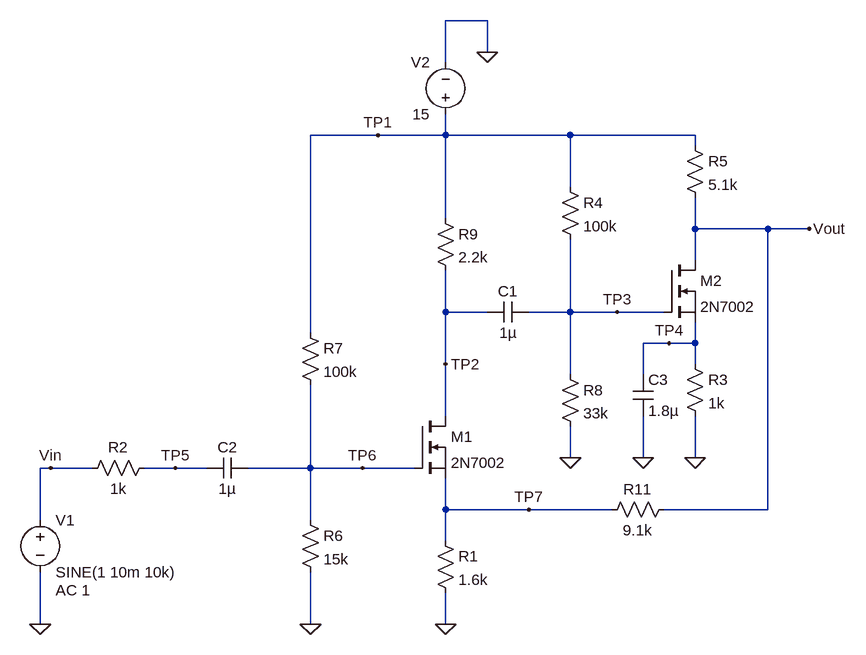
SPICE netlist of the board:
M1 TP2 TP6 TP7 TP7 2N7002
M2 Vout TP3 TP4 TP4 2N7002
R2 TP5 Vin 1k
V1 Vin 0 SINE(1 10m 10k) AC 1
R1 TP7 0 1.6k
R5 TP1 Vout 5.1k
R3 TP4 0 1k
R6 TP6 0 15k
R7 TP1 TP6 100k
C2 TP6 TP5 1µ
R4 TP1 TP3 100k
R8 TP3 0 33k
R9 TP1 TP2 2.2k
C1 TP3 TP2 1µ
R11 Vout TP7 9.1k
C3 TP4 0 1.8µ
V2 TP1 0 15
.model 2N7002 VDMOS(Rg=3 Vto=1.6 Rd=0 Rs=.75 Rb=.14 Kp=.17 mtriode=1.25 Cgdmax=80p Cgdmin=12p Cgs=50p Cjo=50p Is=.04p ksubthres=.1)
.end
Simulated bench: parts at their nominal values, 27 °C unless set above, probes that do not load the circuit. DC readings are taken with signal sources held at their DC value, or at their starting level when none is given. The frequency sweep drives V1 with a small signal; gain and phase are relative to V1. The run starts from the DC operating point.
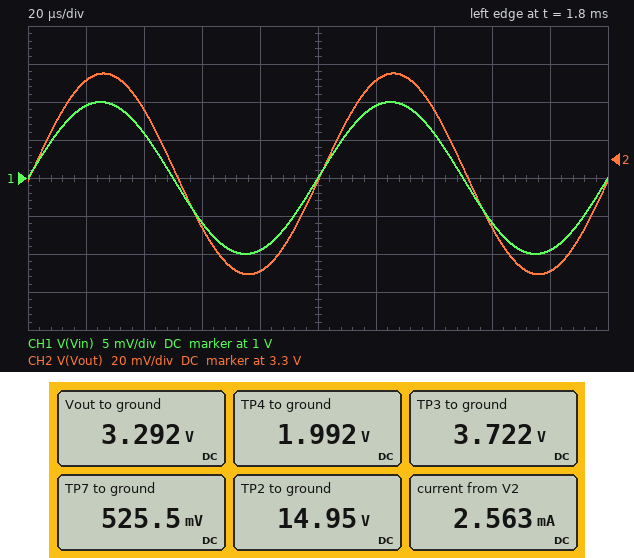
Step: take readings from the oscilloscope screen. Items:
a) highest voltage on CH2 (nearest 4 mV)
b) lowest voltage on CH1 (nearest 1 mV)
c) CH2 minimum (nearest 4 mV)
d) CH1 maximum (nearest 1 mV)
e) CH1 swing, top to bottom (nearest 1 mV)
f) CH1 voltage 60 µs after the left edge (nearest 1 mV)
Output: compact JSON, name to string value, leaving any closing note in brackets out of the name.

{"highest voltage on CH2": "3.344 V", "lowest voltage on CH1": "990 mV", "CH2 minimum": "3.240 V", "CH1 maximum": "1.010 V", "CH1 swing, top to bottom": "20 mV", "CH1 voltage 60 µs after the left edge": "994 mV"}
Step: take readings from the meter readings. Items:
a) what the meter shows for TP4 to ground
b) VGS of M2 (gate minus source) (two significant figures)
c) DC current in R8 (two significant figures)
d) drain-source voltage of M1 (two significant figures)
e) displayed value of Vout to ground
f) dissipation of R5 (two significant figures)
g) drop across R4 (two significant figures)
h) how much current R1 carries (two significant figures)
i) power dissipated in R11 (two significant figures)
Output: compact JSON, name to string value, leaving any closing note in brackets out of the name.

{"what the meter shows for TP4 to ground": "1.992 V", "VGS of M2 (gate minus source)": "1.7 V", "DC current in R8": "110 µA", "drain-source voltage of M1": "14 V", "displayed value of Vout to ground": "3.292 V", "dissipation of R5": "27 mW", "drop across R4": "11 V", "how much current R1 carries": "330 µA", "power dissipated in R11": "840 µW"}
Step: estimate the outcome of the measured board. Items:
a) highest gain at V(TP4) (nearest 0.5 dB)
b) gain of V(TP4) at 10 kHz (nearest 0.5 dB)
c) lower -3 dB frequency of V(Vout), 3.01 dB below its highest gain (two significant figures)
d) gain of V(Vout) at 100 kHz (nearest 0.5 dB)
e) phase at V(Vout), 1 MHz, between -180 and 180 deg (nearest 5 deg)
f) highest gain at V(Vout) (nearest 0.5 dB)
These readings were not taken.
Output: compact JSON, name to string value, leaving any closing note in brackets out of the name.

{"highest gain at V(TP4)": "-8.5 dB", "gain of V(TP4) at 10 kHz": "-37.5 dB", "lower -3 dB frequency of V(Vout), 3.01 dB below its highest gain": "320 Hz", "gain of V(Vout) at 100 kHz": "12.0 dB", "phase at V(Vout), 1 MHz, between -180 and 180 deg": "-135 deg", "highest gain at V(Vout)": "14.5 dB"}
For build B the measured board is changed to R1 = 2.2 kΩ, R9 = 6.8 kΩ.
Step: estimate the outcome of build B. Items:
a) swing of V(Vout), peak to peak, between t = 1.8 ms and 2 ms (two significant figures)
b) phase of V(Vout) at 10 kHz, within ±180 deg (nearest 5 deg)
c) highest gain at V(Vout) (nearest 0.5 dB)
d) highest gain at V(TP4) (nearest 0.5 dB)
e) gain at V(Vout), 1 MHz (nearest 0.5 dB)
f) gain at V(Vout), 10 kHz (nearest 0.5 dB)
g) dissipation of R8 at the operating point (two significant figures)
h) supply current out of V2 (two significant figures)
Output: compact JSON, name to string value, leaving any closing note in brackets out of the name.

{"swing of V(Vout), peak to peak, between t = 1.8 ms and 2 ms": "66 mV", "phase of V(Vout) at 10 kHz, within ±180 deg": "-20 deg", "highest gain at V(Vout)": "11.0 dB", "highest gain at V(TP4)": "-16.0 dB", "gain at V(Vout), 1 MHz": "-12.0 dB", "gain at V(Vout), 10 kHz": "10.5 dB", "dissipation of R8 at the operating point": "420 µW", "supply current out of V2": "2.5 mA"}
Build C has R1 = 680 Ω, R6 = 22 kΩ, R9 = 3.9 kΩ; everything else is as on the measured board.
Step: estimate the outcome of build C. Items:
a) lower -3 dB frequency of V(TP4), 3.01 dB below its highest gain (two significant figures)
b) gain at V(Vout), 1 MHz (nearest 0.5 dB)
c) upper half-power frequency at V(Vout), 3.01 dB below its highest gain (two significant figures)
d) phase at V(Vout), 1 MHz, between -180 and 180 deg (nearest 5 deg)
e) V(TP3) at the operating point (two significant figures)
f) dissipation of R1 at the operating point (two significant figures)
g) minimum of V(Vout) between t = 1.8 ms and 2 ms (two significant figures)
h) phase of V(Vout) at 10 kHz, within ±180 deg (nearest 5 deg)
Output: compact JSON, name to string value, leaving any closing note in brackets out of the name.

{"lower -3 dB frequency of V(TP4), 3.01 dB below its highest gain": "8.4 Hz", "gain at V(Vout), 1 MHz": "10.5 dB", "upper half-power frequency at V(Vout), 3.01 dB below its highest gain": "270 kHz", "phase at V(Vout), 1 MHz, between -180 and 180 deg": "-90 deg", "V(TP3) at the operating point": "3.7 V", "dissipation of R1 at the operating point": "1.5 mW", "minimum of V(Vout) between t = 1.8 ms and 2 ms": "3.3 V", "phase of V(Vout) at 10 kHz, within ±180 deg": "0 deg"}
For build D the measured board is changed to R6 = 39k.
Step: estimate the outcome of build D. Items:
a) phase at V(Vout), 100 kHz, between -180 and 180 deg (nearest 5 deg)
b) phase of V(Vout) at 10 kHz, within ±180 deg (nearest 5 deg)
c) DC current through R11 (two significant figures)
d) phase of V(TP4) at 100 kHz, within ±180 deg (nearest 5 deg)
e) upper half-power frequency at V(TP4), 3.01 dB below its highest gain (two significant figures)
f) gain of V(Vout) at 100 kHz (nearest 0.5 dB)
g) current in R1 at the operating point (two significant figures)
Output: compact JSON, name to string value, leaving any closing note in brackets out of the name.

{"phase at V(Vout), 100 kHz, between -180 and 180 deg": "-15 deg", "phase of V(Vout) at 10 kHz, within ±180 deg": "0 deg", "DC current through R11": "160 µA", "phase of V(TP4) at 100 kHz, within ±180 deg": "80 deg", "upper half-power frequency at V(TP4), 3.01 dB below its highest gain": "220 Hz", "gain of V(Vout) at 100 kHz": "15.5 dB", "current in R1 at the operating point": "1.6 mA"}
